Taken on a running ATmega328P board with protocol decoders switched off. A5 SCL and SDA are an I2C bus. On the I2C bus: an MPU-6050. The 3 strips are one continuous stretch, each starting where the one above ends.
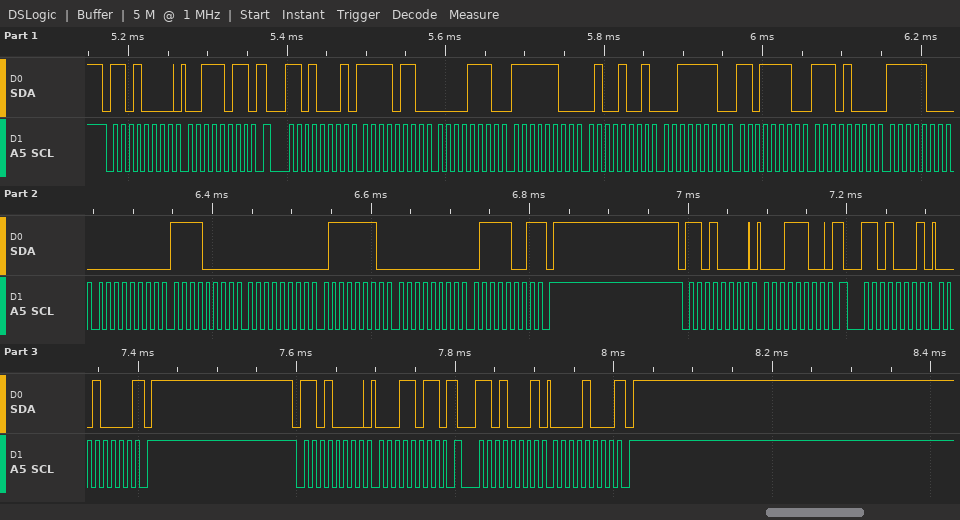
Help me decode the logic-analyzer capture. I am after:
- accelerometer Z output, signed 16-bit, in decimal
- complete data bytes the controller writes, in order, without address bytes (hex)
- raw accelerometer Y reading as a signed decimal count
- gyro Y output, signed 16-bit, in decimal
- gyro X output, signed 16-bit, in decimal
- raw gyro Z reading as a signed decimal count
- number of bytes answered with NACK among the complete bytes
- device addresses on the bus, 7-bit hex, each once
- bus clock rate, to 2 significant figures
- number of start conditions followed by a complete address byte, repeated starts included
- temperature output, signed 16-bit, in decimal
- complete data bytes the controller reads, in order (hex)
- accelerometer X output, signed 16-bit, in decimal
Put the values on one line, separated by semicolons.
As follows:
16094; 3B 1C 1B; -951; 126; 240; 121; 3; 0x68; 100 kHz; 6; -5896; F6 0E FC 49 3E DE E8 F8 00 F0 00 7E 00 79 10 08; -2546
